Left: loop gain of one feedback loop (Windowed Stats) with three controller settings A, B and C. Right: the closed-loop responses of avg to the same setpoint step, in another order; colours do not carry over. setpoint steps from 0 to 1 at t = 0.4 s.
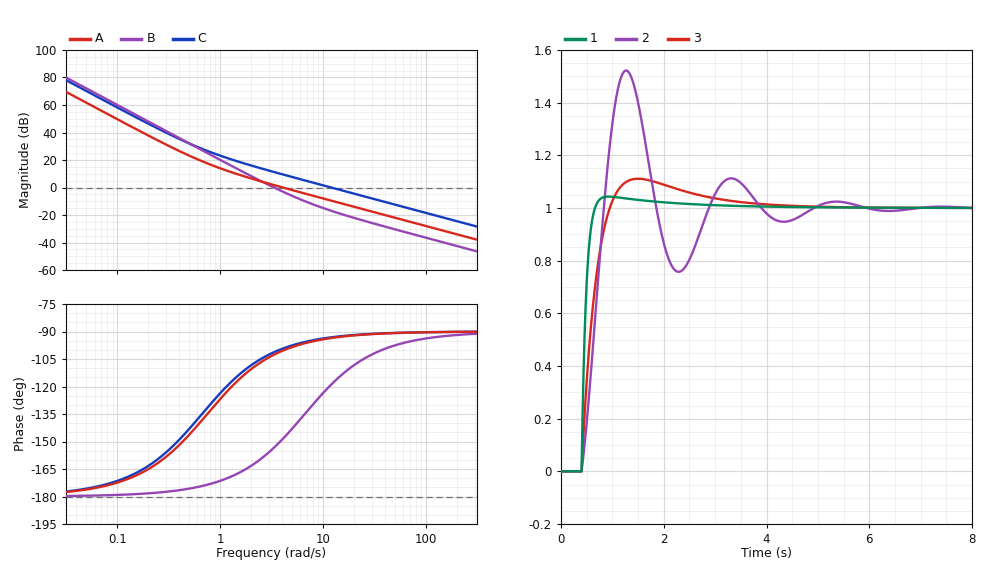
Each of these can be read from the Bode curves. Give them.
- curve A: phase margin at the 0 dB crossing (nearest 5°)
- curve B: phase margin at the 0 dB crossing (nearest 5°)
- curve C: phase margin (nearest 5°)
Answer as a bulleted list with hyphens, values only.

- 80°
- 25°
- 85°
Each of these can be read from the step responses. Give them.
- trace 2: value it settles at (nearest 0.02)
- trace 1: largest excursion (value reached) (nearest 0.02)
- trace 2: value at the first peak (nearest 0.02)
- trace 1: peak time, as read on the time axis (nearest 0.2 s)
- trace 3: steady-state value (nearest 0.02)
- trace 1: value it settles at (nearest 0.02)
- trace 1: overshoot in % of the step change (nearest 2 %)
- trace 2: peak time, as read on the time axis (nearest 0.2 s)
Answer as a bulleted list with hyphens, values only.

- 1.00
- 1.04
- 1.52
- 1.0 s
- 1.00
- 1.00
- 4 %
- 1.2 s
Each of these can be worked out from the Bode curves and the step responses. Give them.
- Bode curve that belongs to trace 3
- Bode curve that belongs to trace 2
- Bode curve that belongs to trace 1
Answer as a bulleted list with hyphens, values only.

- A
- B
- C
